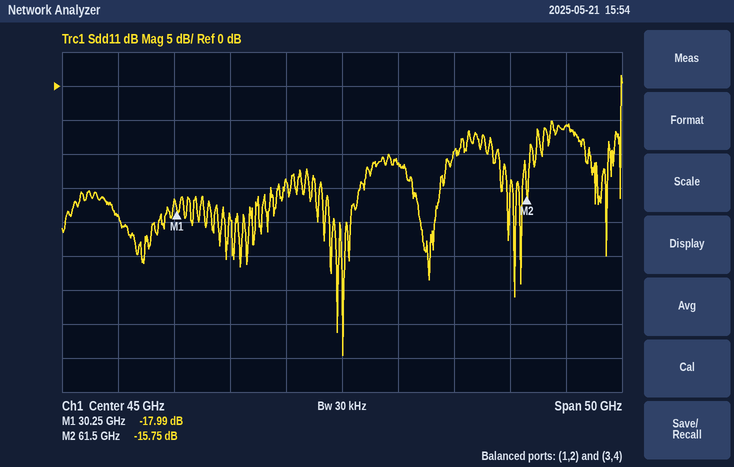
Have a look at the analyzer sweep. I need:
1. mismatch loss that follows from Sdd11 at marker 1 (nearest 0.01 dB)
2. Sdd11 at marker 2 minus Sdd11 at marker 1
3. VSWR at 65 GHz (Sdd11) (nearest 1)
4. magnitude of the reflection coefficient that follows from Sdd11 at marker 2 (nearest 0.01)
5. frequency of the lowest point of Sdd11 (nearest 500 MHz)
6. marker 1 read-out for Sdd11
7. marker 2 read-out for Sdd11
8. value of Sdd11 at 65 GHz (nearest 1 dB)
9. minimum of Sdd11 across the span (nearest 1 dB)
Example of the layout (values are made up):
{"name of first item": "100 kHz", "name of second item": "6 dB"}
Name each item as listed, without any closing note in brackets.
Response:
{"mismatch loss that follows from Sdd11 at marker 1": "0.07 dB", "Sdd11 at marker 2 minus Sdd11 at marker 1": "2.24 dB", "VSWR at 65 GHz (Sdd11)": "3", "magnitude of the reflection coefficient that follows from Sdd11 at marker 2": "0.16", "frequency of the lowest point of Sdd11": "45.0 GHz", "marker 1 read-out for Sdd11": "-17.99 dB", "marker 2 read-out for Sdd11": "-15.75 dB", "value of Sdd11 at 65 GHz": "-6 dB", "minimum of Sdd11 across the span": "-40 dB"}
